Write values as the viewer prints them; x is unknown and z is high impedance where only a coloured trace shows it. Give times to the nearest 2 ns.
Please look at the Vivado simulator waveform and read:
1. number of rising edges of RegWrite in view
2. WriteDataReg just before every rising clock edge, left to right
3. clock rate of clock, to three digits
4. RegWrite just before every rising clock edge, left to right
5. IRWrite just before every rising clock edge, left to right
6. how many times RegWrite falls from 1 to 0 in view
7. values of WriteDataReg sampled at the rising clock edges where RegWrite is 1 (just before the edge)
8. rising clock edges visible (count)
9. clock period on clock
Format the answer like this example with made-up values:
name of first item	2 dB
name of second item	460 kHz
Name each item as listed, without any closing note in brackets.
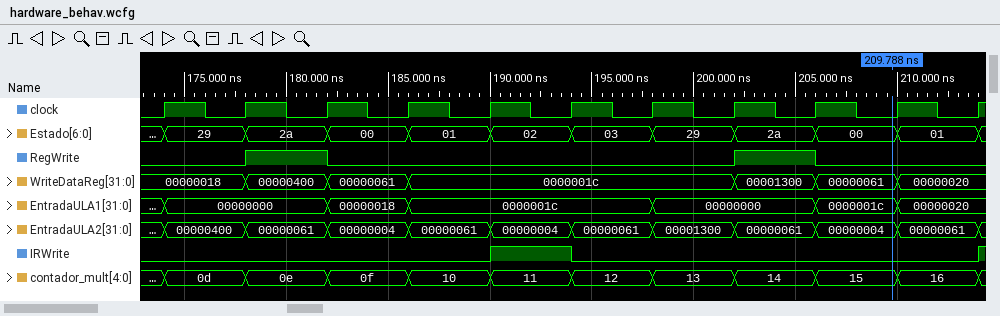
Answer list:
number of rising edges of RegWrite in view	2
WriteDataReg just before every rising clock edge, left to right	00000018, 00000018, 00000400, 00000061, 0000001c, 0000001c, 0000001c, 0000001c, 00001300, 00000061, 00000020
clock rate of clock, to three digits	250 MHz
RegWrite just before every rising clock edge, left to right	0 0 1 0 0 0 0 0 1 0 0
IRWrite just before every rising clock edge, left to right	0 0 0 0 0 1 0 0 0 0 0
how many times RegWrite falls from 1 to 0 in view	2
values of WriteDataReg sampled at the rising clock edges where RegWrite is 1	00000400, 00001300
rising clock edges visible	11
clock period on clock	4 ns
